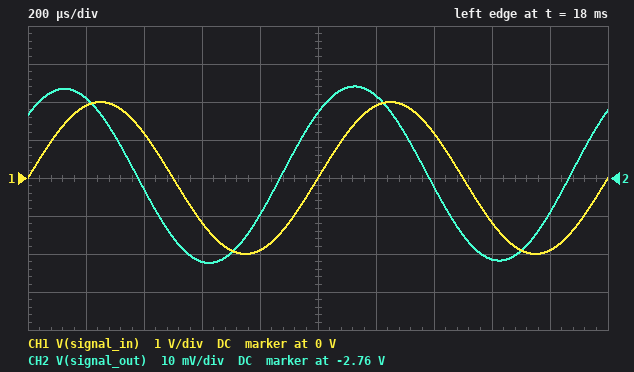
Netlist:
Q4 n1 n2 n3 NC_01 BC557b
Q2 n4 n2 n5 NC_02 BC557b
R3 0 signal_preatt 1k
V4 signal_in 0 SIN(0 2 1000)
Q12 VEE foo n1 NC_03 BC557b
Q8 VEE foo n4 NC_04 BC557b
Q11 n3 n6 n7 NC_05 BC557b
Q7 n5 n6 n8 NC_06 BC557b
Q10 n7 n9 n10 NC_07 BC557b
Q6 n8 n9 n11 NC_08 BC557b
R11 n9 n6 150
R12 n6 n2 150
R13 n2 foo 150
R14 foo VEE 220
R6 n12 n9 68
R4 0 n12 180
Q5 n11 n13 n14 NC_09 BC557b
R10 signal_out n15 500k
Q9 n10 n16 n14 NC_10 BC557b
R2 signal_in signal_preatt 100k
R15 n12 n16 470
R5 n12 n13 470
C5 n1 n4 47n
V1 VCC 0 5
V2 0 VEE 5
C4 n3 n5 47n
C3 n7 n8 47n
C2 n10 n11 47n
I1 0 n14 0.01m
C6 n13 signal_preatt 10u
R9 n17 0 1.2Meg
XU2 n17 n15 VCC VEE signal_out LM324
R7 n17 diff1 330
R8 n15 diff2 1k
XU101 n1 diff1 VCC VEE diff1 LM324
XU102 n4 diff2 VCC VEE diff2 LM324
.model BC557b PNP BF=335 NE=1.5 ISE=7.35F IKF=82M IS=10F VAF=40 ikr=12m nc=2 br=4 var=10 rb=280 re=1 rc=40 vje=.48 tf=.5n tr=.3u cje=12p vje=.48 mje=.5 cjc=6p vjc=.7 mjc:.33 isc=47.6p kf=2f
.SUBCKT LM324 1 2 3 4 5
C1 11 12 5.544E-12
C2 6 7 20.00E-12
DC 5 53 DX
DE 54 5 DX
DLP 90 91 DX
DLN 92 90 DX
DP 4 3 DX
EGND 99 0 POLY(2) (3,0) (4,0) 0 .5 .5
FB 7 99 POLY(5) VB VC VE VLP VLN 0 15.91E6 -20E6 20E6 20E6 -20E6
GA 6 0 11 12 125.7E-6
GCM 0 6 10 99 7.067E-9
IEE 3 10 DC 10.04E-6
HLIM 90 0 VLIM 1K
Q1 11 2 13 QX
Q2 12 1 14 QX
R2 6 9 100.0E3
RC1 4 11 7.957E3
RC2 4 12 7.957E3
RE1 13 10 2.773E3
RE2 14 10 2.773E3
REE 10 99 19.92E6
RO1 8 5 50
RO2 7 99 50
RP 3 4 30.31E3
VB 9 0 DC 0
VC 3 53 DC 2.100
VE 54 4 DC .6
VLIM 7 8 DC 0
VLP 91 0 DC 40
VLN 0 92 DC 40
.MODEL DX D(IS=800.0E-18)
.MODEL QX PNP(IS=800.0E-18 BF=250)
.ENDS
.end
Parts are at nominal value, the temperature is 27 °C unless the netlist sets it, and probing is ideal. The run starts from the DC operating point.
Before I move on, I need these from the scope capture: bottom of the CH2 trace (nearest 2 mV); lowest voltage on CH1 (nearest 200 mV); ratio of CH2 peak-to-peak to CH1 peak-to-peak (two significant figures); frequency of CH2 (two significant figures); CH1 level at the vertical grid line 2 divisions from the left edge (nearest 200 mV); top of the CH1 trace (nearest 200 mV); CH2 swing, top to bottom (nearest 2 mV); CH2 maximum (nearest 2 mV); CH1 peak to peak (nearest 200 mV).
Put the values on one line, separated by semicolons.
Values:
-2.782 V; -2.0 V; 0.012; 1.0 kHz; 1.2 V; 2.0 V; 46 mV; -2.736 V; 4.0 V
